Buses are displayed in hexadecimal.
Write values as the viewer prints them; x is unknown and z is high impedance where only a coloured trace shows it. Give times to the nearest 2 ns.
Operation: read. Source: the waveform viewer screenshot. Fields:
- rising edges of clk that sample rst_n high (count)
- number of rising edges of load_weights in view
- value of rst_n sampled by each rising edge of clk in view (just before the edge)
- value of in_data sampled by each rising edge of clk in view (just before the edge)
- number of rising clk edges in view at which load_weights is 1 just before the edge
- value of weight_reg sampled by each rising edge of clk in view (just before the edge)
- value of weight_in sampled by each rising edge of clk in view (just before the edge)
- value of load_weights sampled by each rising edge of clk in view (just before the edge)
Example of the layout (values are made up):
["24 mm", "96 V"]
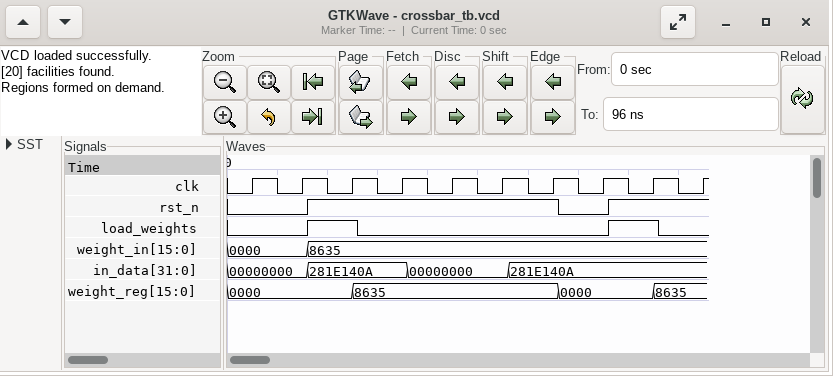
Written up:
["7", "2", "0 0 1 1 1 1 1 0 1 1", "00000000, 00000000, 281E140A, 281E140A, 00000000, 00000000, 281E140A, 281E140A, 281E140A, 281E140A", "2", "0000, 0000, 0000, 8635, 8635, 8635, 8635, 0000, 0000, 8635", "0000, 0000, 8635, 8635, 8635, 8635, 8635, 8635, 8635, 8635", "0 0 1 0 0 0 0 0 1 0"]
